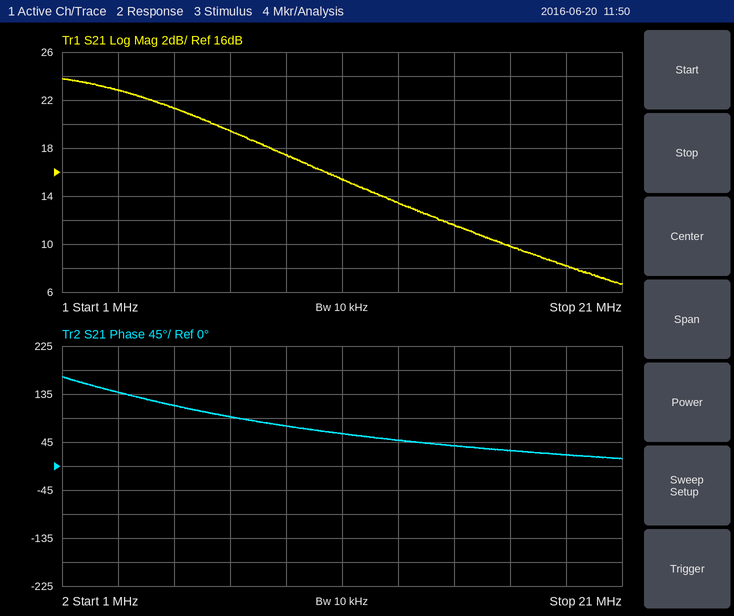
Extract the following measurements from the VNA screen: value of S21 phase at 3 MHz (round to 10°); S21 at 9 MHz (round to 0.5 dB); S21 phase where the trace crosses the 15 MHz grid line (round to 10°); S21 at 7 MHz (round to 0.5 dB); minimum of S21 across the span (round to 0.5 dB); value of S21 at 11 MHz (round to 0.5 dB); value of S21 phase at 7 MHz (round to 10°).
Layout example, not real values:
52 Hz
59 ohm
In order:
140°
17.5 dB
40°
19.5 dB
6.5 dB
15.5 dB
90°
